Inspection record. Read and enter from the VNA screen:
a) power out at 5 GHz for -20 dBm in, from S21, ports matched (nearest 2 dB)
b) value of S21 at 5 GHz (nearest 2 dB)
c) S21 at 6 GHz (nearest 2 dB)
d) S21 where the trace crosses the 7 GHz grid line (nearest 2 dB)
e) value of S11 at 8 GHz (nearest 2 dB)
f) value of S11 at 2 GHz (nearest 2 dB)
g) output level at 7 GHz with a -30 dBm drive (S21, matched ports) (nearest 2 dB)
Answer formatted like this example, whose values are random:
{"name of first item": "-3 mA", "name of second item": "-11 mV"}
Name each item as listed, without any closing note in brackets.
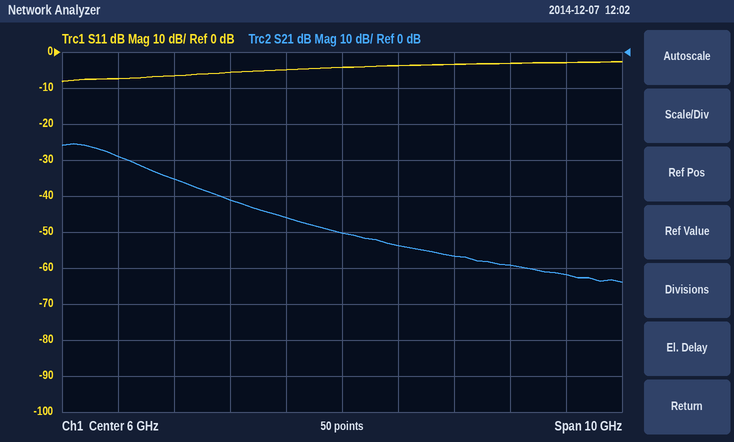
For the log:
{"power out at 5 GHz for -20 dBm in, from S21, ports matched": "-66 dBm", "value of S21 at 5 GHz": "-46 dB", "S21 at 6 GHz": "-50 dB", "S21 where the trace crosses the 7 GHz grid line": "-54 dB", "value of S11 at 8 GHz": "-4 dB", "value of S11 at 2 GHz": "-8 dB", "output level at 7 GHz with a -30 dBm drive (S21, matched ports)": "-84 dBm"}
